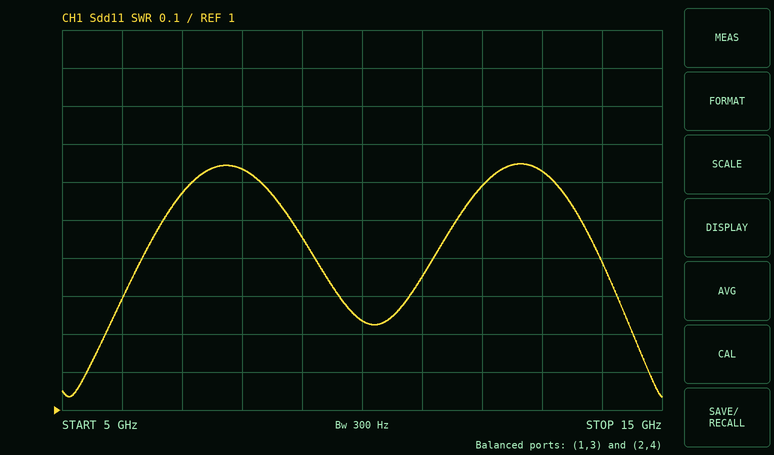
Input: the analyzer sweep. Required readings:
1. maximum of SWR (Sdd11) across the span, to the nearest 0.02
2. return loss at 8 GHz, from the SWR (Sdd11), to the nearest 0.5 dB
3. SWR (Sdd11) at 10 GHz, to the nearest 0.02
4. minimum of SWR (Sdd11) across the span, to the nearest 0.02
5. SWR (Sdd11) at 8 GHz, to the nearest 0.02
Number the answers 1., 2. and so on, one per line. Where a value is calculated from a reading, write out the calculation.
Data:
1. 1.64
2. −20 log10((1.64 − 1)/(1.64 + 1)) ≈ 12.3 dB, so 12.5 dB to the nearest 0.5 dB
3. 1.24
4. 1.04
5. 1.64
